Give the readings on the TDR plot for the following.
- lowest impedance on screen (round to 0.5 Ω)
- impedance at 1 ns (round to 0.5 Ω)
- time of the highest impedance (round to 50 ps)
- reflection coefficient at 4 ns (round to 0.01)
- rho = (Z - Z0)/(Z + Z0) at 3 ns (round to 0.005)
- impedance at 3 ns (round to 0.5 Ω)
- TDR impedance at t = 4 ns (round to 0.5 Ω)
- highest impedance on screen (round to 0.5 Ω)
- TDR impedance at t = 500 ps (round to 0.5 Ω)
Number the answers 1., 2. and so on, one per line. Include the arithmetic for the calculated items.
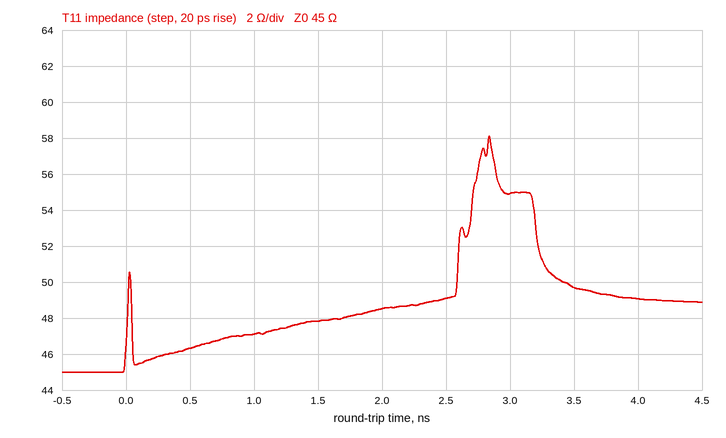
1. 45.0 Ω
2. 47.0 Ω
3. 2.85 ns
4. (49 − 45)/(49 + 45) ≈ +0.04
5. (55 − 45)/(55 + 45) ≈ +0.100
6. 55.0 Ω
7. 49.0 Ω
8. 58.0 Ω
9. 46.5 Ω
